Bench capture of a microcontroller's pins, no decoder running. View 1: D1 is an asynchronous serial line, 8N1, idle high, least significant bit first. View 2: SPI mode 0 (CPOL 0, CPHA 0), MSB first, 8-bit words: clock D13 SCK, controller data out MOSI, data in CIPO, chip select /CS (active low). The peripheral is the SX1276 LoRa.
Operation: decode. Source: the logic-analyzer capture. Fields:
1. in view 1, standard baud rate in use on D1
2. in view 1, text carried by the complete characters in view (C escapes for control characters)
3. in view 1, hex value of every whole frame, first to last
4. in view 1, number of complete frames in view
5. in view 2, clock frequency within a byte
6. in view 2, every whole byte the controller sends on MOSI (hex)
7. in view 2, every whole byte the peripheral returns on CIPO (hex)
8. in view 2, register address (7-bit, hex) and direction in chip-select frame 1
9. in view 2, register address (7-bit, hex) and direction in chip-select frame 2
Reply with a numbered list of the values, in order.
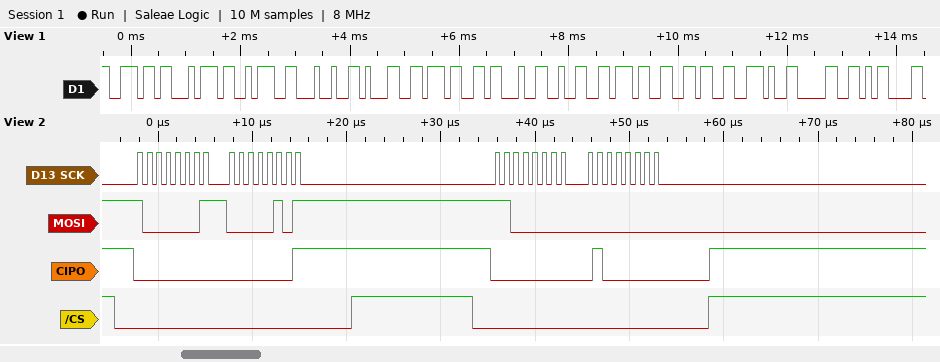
1. 9600 baud
2. "nt:$17#276.0\r"
3. 0x6E 0x74 0x3A 0x24 0x31 0x37 0x23 0x32 0x37 0x36 0x2E 0x30 0x0D
4. 13
5. 1 MHz
6. 0x81 0x05 0xC0 0x00
7. 0x00 0x01 0x00 0x40
8. 0x01 write
9. 0x40 write
